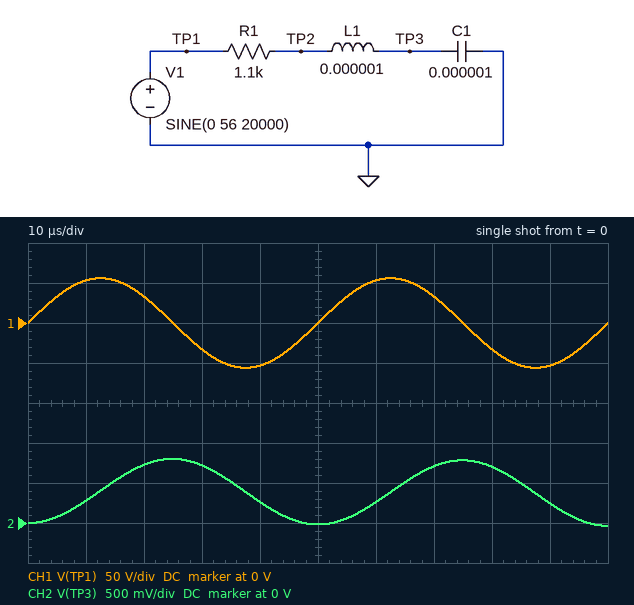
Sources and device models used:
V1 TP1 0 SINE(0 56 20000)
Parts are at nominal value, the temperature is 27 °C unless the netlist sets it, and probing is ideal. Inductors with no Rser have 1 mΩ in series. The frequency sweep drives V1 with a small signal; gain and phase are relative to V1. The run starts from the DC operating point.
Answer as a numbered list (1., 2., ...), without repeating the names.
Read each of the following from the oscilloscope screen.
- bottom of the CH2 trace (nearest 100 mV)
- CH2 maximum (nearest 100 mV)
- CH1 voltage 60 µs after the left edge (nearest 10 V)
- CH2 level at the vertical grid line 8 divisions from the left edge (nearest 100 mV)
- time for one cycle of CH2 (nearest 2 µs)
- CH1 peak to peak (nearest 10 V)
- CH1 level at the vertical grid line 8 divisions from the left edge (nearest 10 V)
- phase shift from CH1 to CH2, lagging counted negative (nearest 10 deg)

1. 0 V
2. 800 mV
3. 50 V
4. 700 mV
5. 50 µs
6. 110 V
7. -30 V
8. -90 deg
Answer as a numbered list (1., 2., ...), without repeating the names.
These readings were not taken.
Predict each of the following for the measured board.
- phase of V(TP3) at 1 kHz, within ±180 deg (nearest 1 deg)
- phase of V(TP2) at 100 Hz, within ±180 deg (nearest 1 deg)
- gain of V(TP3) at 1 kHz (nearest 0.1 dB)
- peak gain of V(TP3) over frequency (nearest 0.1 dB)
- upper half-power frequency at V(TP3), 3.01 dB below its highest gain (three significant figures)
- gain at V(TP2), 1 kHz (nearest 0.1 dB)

1. -82 deg
2. -35 deg
3. -16.9 dB
4. 0 dB
5. 145 Hz
6. -16.9 dB
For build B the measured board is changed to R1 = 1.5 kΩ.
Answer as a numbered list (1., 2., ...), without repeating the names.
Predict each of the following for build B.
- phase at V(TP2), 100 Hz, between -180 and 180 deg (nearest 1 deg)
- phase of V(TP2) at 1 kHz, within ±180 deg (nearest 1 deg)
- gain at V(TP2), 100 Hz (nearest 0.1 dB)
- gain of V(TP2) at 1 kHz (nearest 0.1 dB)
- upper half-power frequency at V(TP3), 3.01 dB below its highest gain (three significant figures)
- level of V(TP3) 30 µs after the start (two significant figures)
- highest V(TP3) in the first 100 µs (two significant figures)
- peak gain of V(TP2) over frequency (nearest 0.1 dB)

1. -43 deg
2. -84 deg
3. -2.8 dB
4. -19.5 dB
5. 106 Hz
6. 530 mV
7. 590 mV
8. 0 dB
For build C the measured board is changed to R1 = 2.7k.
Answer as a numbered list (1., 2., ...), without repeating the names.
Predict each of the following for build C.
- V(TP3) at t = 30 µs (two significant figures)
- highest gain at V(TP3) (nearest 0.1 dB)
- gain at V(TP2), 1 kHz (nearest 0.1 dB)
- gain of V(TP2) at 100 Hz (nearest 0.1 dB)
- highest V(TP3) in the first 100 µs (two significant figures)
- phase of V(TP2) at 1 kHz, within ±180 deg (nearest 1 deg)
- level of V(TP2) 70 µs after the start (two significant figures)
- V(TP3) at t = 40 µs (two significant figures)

1. 300 mV
2. 0 dB
3. -24.6 dB
4. -5.9 dB
5. 330 mV
6. -87 deg
7. 290 mV
8. 110 mV
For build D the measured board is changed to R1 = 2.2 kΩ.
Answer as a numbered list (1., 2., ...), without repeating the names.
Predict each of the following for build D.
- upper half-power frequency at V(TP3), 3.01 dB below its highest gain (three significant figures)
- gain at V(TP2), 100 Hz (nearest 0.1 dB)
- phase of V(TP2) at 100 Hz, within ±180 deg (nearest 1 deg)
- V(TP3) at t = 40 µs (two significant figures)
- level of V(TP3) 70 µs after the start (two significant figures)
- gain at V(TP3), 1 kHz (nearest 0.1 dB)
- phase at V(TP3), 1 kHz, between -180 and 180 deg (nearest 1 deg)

1. 72.3 Hz
2. -4.6 dB
3. -54 deg
4. 140 mV
5. 360 mV
6. -22.8 dB
7. -86 deg
